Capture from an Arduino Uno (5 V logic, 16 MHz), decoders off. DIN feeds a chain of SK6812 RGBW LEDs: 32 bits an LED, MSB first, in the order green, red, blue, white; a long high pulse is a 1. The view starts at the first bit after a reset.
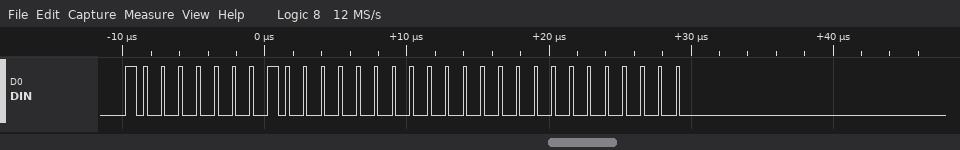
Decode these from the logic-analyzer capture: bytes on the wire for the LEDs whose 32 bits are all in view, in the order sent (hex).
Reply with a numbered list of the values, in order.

1. 80 80 00 00
